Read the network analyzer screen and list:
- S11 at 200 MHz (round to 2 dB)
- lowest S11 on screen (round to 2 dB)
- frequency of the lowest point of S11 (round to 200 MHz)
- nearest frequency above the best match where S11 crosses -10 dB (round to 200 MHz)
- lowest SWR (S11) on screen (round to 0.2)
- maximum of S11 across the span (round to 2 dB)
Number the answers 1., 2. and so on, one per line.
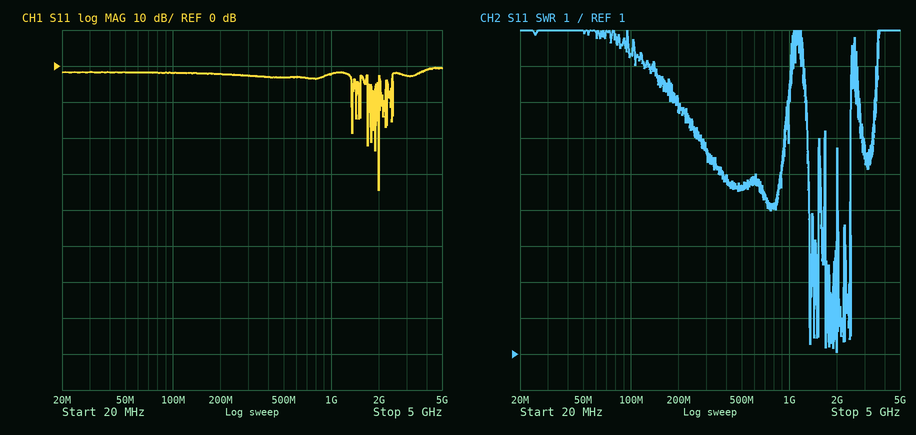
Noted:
1. -2 dB
2. -34 dB
3. 2.0 GHz
4. 2.0 GHz
5. 1.0
6. 0 dB
